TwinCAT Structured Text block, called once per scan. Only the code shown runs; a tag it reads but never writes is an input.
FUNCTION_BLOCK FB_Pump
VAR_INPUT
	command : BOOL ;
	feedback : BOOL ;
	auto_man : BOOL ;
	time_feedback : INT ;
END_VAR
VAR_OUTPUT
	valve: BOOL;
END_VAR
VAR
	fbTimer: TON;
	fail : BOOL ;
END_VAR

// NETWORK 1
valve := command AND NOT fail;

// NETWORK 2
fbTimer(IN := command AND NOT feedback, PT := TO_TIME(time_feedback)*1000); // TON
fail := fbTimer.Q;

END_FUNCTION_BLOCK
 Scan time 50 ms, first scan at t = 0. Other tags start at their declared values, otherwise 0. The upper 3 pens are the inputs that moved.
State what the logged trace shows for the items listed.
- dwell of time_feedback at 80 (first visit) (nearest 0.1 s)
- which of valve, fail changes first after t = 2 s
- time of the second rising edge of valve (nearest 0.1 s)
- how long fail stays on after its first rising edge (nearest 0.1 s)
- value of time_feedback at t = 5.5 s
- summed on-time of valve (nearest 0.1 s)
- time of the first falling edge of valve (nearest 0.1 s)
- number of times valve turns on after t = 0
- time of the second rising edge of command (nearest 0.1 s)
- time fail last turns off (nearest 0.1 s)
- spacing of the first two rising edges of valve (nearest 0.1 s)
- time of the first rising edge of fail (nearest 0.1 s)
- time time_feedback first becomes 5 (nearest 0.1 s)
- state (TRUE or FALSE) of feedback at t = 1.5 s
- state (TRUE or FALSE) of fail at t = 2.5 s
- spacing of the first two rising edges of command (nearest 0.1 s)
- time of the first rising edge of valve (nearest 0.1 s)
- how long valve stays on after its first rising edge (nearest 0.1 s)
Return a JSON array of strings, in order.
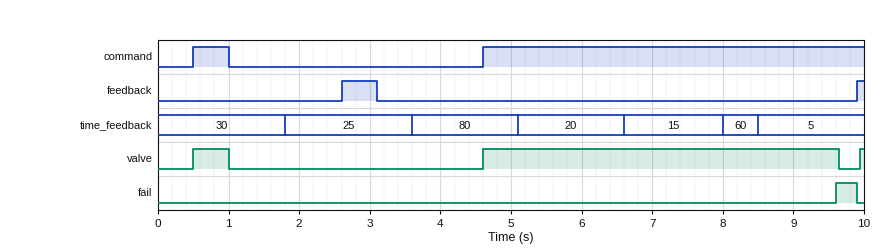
["1.5 s", "valve", "4.6 s", "0.3 s", "20", "5.6 s", "1.0 s", "3", "4.6 s", "9.9 s", "4.1 s", "9.6 s", "8.5 s", "FALSE", "FALSE", "4.1 s", "0.5 s", "0.5 s"]
